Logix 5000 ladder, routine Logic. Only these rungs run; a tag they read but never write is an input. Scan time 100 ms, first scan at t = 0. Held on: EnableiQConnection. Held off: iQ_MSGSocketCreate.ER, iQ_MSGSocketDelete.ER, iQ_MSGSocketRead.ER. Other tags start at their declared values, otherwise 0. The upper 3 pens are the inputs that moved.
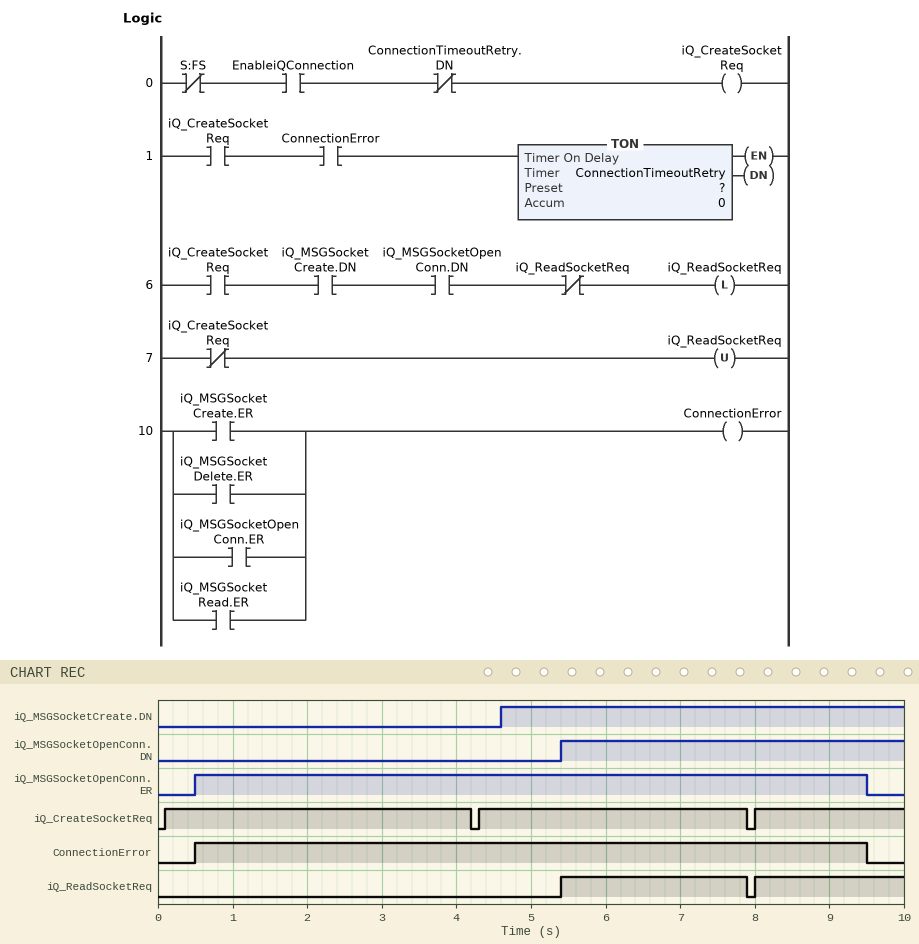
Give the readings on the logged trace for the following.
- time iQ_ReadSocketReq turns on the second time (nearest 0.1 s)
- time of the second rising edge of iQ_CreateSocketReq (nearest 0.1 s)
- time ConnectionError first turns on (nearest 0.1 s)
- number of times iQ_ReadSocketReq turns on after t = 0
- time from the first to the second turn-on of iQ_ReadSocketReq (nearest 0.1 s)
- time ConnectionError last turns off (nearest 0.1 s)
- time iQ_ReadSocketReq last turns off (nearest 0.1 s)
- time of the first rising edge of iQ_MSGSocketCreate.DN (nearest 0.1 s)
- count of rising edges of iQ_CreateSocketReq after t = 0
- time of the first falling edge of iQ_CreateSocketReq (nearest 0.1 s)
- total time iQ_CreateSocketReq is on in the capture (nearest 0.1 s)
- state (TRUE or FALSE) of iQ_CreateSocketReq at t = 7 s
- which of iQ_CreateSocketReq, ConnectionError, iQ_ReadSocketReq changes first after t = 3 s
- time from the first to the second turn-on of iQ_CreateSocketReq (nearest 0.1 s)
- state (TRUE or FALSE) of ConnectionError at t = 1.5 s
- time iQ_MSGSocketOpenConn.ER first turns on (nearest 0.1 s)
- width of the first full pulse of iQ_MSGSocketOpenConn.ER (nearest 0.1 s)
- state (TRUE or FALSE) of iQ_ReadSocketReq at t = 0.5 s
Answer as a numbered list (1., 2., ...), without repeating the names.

1. 8.0 s
2. 4.3 s
3. 0.5 s
4. 2
5. 2.6 s
6. 9.5 s
7. 7.9 s
8. 4.6 s
9. 3
10. 4.2 s
11. 9.7 s
12. TRUE
13. iQ_CreateSocketReq
14. 4.2 s
15. TRUE
16. 0.5 s
17. 9.0 s
18. FALSE
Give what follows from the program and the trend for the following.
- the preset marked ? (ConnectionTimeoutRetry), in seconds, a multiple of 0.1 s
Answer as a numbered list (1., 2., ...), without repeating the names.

1. 3.5 s
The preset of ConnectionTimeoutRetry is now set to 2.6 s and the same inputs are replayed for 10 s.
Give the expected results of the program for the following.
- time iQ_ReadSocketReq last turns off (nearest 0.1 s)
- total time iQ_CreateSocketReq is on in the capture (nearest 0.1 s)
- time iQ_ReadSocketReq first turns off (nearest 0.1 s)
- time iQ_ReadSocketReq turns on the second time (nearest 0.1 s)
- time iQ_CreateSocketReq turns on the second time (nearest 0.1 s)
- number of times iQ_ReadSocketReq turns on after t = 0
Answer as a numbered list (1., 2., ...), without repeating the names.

1. 8.9 s
2. 9.6 s
3. 6.1 s
4. 6.2 s
5. 3.4 s
6. 3
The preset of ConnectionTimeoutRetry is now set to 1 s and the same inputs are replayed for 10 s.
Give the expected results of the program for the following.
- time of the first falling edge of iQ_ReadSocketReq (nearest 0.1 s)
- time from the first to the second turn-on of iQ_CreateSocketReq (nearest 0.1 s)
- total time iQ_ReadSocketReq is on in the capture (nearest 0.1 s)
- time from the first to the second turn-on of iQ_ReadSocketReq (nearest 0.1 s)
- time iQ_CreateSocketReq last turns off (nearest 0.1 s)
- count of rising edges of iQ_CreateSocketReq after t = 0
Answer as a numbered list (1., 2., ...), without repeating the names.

1. 6.5 s
2. 1.7 s
3. 4.3 s
4. 1.2 s
5. 8.9 s
6. 8
